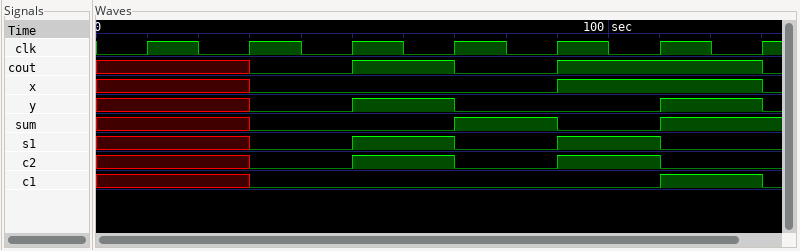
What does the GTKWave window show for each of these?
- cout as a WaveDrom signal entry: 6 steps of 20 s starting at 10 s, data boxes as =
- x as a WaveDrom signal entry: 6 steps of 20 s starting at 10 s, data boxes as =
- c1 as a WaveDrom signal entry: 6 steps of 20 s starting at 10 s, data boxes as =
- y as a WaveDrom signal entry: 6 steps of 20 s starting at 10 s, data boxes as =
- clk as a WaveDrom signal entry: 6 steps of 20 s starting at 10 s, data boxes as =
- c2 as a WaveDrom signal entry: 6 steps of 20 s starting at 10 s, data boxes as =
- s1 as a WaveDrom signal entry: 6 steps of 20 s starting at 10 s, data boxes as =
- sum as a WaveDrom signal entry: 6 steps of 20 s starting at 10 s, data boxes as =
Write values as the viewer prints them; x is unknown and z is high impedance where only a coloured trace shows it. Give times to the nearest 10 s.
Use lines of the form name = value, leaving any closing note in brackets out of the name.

cout as a WaveDrom signal entry: 6 steps of 20 s starting at 10 s, data boxes as = = {name: 'cout', wave: 'x0101.'}
x as a WaveDrom signal entry: 6 steps of 20 s starting at 10 s, data boxes as = = {name: 'x', wave: 'x0..1.'}
c1 as a WaveDrom signal entry: 6 steps of 20 s starting at 10 s, data boxes as = = {name: 'c1', wave: 'x0...1'}
y as a WaveDrom signal entry: 6 steps of 20 s starting at 10 s, data boxes as = = {name: 'y', wave: 'x010.1'}
clk as a WaveDrom signal entry: 6 steps of 20 s starting at 10 s, data boxes as = = {name: 'clk', wave: 'p.....'}
c2 as a WaveDrom signal entry: 6 steps of 20 s starting at 10 s, data boxes as = = {name: 'c2', wave: 'x01010'}
s1 as a WaveDrom signal entry: 6 steps of 20 s starting at 10 s, data boxes as = = {name: 's1', wave: 'x01010'}
sum as a WaveDrom signal entry: 6 steps of 20 s starting at 10 s, data boxes as = = {name: 'sum', wave: 'x0.101'}
